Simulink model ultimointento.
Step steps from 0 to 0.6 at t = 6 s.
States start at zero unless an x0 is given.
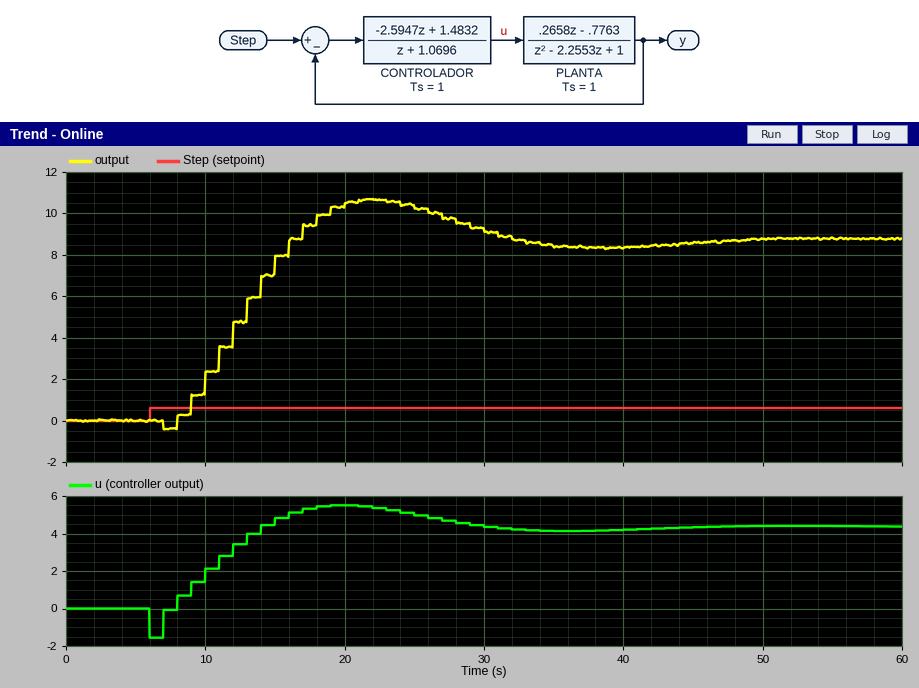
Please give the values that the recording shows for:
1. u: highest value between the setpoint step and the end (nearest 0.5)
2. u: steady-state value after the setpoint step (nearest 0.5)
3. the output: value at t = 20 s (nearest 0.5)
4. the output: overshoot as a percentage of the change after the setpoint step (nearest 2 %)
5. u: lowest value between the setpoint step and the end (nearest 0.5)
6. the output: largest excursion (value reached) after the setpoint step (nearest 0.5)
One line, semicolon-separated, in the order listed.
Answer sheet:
5.5; 4.5; 10.5; 22 %; -1.5; 10.5
